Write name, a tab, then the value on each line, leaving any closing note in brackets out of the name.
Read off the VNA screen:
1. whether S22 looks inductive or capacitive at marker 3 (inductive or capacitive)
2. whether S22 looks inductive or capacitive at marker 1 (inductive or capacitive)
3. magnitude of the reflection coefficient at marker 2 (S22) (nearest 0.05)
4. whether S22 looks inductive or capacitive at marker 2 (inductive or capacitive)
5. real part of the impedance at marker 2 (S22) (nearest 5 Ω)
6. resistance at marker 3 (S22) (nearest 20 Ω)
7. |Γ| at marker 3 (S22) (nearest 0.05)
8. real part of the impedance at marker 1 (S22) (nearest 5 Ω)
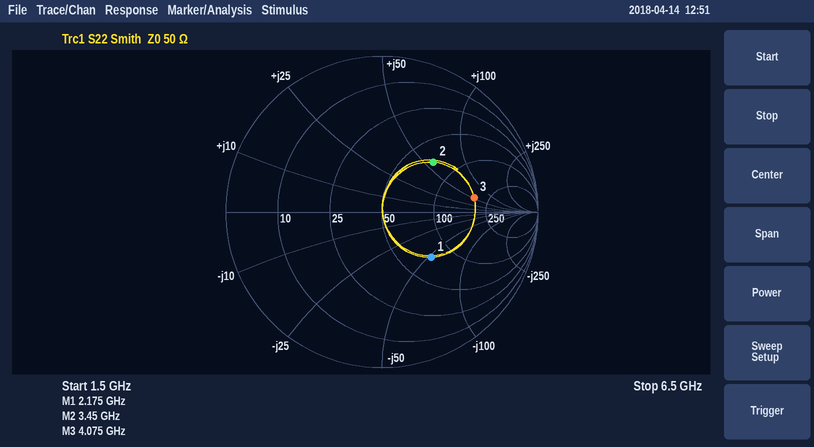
whether S22 looks inductive or capacitive at marker 3	inductive
whether S22 looks inductive or capacitive at marker 1	capacitive
magnitude of the reflection coefficient at marker 2 (S22)	0.45
whether S22 looks inductive or capacitive at marker 2	inductive
real part of the impedance at marker 2 (S22)	70 Ω
resistance at marker 3 (S22)	180 Ω
|Γ| at marker 3 (S22)	0.60
real part of the impedance at marker 1 (S22)	75 Ω
